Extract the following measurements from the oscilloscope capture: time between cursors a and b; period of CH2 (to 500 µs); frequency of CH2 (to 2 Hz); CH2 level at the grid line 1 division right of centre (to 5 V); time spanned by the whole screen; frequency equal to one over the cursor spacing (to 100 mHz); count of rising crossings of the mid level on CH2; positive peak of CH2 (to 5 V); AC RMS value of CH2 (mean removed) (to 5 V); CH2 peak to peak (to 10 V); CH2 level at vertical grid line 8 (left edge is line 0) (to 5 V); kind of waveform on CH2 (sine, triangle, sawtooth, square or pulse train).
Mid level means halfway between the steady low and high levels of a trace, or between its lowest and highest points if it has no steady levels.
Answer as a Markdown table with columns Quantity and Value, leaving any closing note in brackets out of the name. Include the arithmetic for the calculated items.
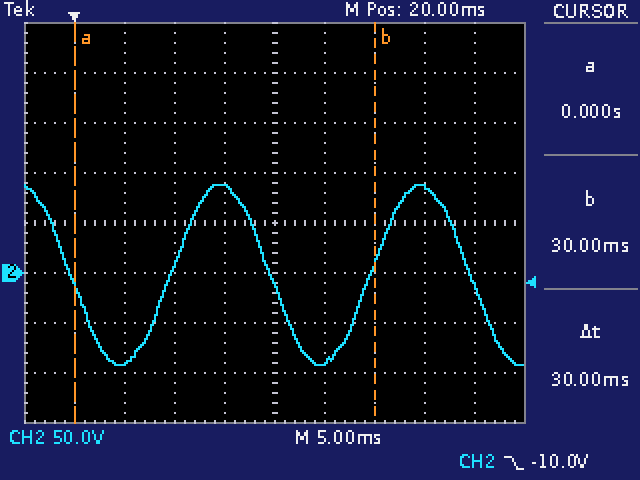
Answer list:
| Quantity | Value |
|---|---|
| time between cursors a and b | 30 ms |
| period of CH2 | 20.0 ms |
| frequency of CH2 | 1 / 20.0 ms ≈ 50 Hz |
| CH2 level at the grid line 1 division right of centre | -90 V |
| time spanned by the whole screen | 50 ms |
| frequency equal to one over the cursor spacing | 1 / 30 ms ≈ 33.3 Hz |
| count of rising crossings of the mid level on CH2 | 2 |
| positive peak of CH2 | 90 V |
| AC RMS value of CH2 (mean removed) | 180 V / (2√2) ≈ 63.6 V, so 65 V to the nearest 5 V |
| CH2 peak to peak | 180 V |
| CH2 level at vertical grid line 8 (left edge is line 0) | 85 V |
| kind of waveform on CH2 | sine |
